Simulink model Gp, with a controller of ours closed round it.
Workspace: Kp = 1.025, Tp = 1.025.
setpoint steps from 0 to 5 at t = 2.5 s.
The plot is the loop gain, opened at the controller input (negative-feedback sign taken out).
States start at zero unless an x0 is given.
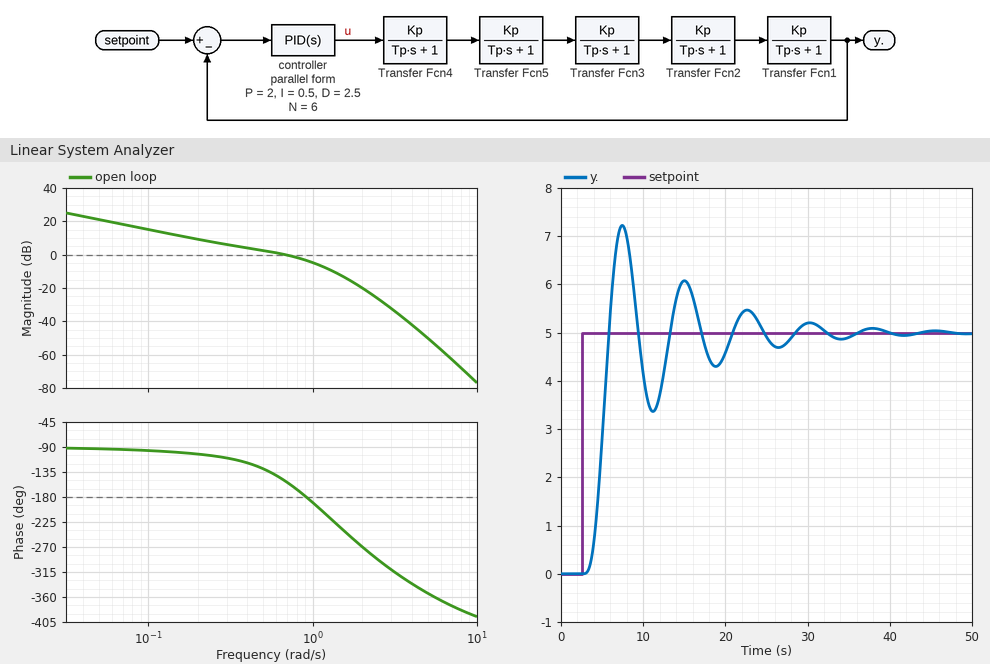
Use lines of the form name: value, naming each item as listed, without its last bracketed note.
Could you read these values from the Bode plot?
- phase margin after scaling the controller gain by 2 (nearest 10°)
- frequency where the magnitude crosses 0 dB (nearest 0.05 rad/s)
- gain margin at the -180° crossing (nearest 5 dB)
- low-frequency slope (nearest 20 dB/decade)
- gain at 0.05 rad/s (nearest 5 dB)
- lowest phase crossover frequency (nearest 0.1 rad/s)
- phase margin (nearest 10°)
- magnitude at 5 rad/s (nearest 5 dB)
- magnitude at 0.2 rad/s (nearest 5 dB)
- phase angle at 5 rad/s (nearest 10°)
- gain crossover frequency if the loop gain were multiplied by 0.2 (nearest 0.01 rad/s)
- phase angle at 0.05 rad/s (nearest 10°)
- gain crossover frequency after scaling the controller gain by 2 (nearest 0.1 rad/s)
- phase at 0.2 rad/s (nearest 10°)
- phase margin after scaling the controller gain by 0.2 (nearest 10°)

phase margin after scaling the controller gain by 2: -20°
frequency where the magnitude crosses 0 dB: 0.70 rad/s
gain margin at the -180° crossing: 5 dB
low-frequency slope: -20 dB/decade
gain at 0.05 rad/s: 20 dB
lowest phase crossover frequency: 0.9 rad/s
phase margin: 30°
magnitude at 5 rad/s: -50 dB
magnitude at 0.2 rad/s: 10 dB
phase angle at 5 rad/s: -350°
gain crossover frequency if the loop gain were multiplied by 0.2: 0.11 rad/s
phase angle at 0.05 rad/s: -90°
gain crossover frequency after scaling the controller gain by 2: 1.1 rad/s
phase at 0.2 rad/s: -100°
phase margin after scaling the controller gain by 0.2: 80°
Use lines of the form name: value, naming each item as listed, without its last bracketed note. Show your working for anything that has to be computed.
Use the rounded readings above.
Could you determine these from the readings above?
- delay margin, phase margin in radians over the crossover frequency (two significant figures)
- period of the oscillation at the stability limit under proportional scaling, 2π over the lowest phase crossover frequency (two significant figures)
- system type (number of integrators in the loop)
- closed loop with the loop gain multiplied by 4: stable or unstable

delay margin, phase margin in radians over the crossover frequency: 30 × π / 180 / 0.7 = 0.75 s
period of the oscillation at the stability limit under proportional scaling, 2π over the lowest phase crossover frequency: 2π / 0.9 = 7.0 s
system type: 1
closed loop with the loop gain multiplied by 4: stable or unstable: unstable
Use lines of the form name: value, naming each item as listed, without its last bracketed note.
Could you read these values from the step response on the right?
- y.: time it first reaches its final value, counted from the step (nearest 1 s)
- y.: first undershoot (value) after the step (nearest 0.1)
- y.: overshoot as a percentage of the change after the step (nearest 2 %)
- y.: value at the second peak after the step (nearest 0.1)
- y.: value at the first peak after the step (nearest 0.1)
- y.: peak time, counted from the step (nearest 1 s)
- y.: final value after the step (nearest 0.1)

y.: time it first reaches its final value, counted from the step: 3 s
y.: first undershoot (value) after the step: 3.4
y.: overshoot as a percentage of the change after the step: 44 %
y.: value at the second peak after the step: 6.1
y.: value at the first peak after the step: 7.2
y.: peak time, counted from the step: 5 s
y.: final value after the step: 5.0
